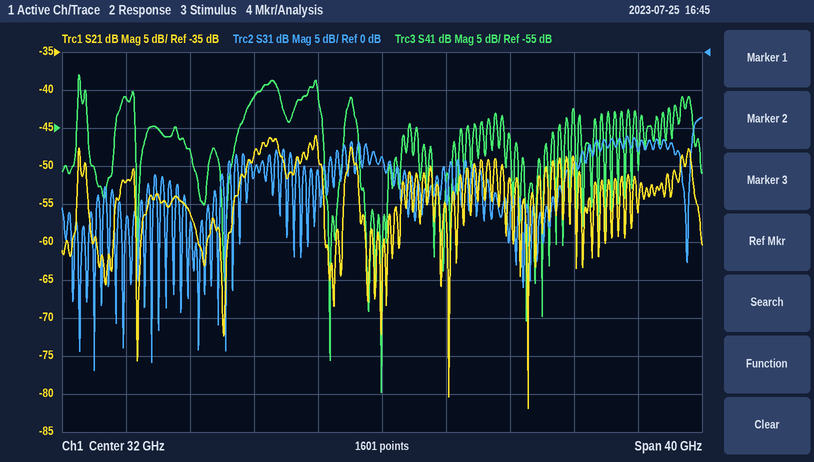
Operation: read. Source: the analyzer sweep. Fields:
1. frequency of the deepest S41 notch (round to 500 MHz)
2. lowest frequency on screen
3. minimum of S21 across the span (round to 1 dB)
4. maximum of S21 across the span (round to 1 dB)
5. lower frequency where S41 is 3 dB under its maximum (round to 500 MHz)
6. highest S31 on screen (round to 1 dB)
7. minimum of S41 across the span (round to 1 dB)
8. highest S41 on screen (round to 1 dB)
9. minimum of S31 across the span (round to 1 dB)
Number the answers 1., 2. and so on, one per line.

1. 32.0 GHz
2. 12 GHz
3. -82 dB
4. -46 dB
5. 13.0 GHz
6. -9 dB
7. -90 dB
8. -48 dB
9. -42 dB
